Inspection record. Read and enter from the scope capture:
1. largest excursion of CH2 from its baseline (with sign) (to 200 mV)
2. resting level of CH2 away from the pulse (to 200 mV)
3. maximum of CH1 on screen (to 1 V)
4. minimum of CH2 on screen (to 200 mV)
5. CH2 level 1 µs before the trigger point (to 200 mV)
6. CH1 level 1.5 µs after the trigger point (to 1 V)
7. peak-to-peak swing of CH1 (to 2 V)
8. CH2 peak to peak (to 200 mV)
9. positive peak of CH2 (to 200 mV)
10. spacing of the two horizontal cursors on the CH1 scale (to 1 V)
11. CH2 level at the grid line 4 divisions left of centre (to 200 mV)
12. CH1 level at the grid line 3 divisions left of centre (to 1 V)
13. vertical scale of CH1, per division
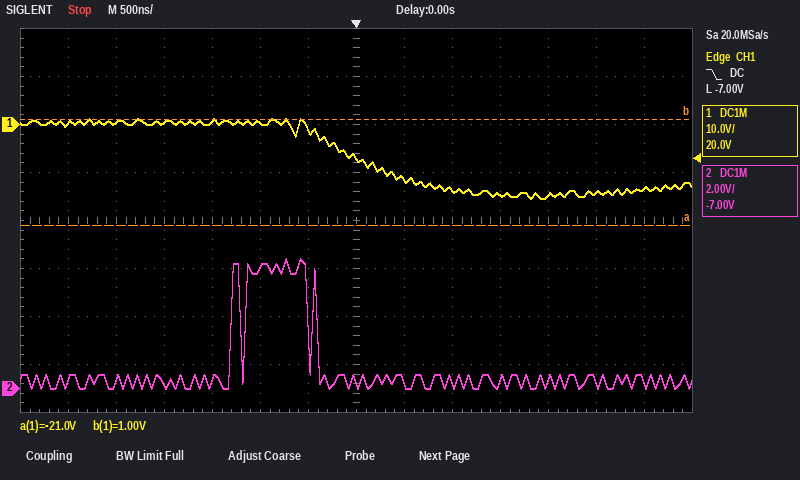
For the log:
+5.0 V
400 mV
1 V
0.0 V
5.0 V
-15 V
16 V
5.4 V
5.4 V
22 V
200 mV
1 V
10 V
